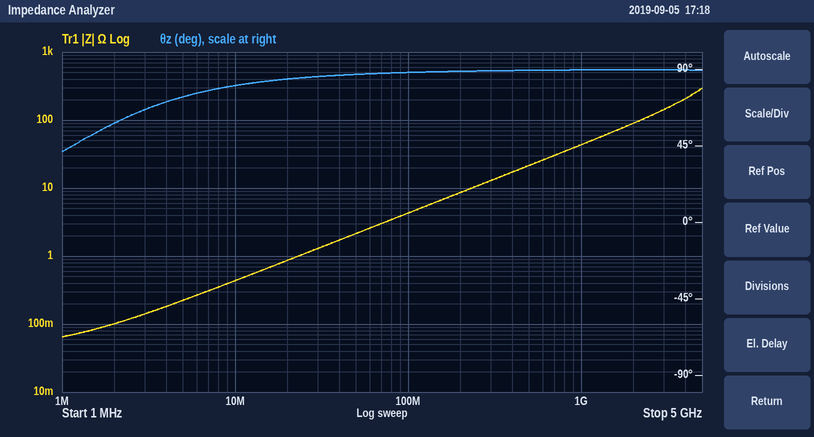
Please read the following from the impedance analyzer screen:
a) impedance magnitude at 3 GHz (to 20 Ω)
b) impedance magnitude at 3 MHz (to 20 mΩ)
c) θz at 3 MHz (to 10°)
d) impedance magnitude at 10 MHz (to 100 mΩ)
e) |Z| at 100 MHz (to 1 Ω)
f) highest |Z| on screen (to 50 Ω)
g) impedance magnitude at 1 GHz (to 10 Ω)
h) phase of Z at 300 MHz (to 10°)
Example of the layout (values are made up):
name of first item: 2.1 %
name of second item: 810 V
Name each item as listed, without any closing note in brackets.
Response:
impedance magnitude at 3 GHz: 140 Ω
impedance magnitude at 3 MHz: 140 mΩ
θz at 3 MHz: 70°
impedance magnitude at 10 MHz: 400 mΩ
|Z| at 100 MHz: 4 Ω
highest |Z| on screen: 300 Ω
impedance magnitude at 1 GHz: 40 Ω
phase of Z at 300 MHz: 90°
